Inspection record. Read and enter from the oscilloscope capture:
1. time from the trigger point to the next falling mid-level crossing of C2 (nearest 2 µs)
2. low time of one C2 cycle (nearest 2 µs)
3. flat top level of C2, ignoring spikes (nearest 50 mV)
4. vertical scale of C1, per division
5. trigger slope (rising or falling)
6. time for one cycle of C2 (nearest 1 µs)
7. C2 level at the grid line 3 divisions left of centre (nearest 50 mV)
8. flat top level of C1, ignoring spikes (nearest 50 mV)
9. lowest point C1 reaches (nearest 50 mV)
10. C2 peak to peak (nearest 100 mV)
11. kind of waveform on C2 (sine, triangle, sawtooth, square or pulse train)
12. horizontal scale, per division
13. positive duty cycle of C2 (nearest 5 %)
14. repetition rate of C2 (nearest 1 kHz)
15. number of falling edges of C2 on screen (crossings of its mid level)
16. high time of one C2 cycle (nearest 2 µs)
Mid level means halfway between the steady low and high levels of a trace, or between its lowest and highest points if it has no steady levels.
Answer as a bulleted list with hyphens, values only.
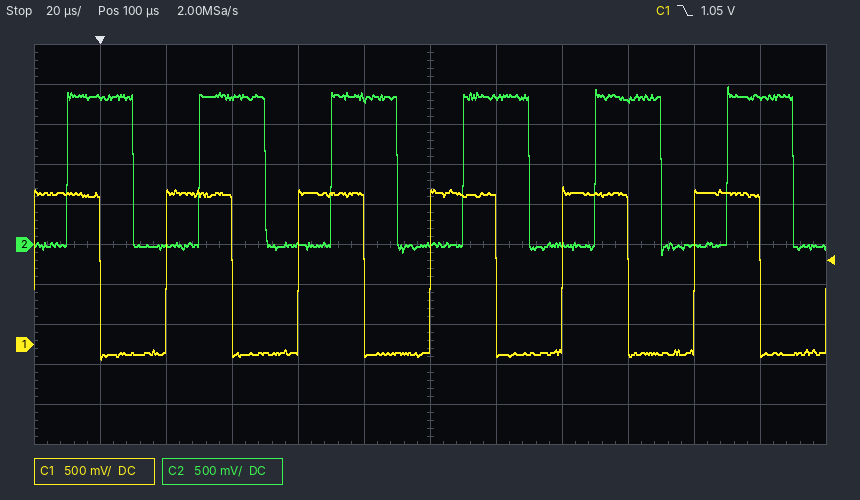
- 10 µs
- 20 µs
- 1.85 V
- 500 mV
- falling
- 40 µs
- 1.85 V
- 1.90 V
- -200 mV
- 2.10 V
- square
- 20 µs
- 50 %
- 25 kHz
- 6
- 20 µs
